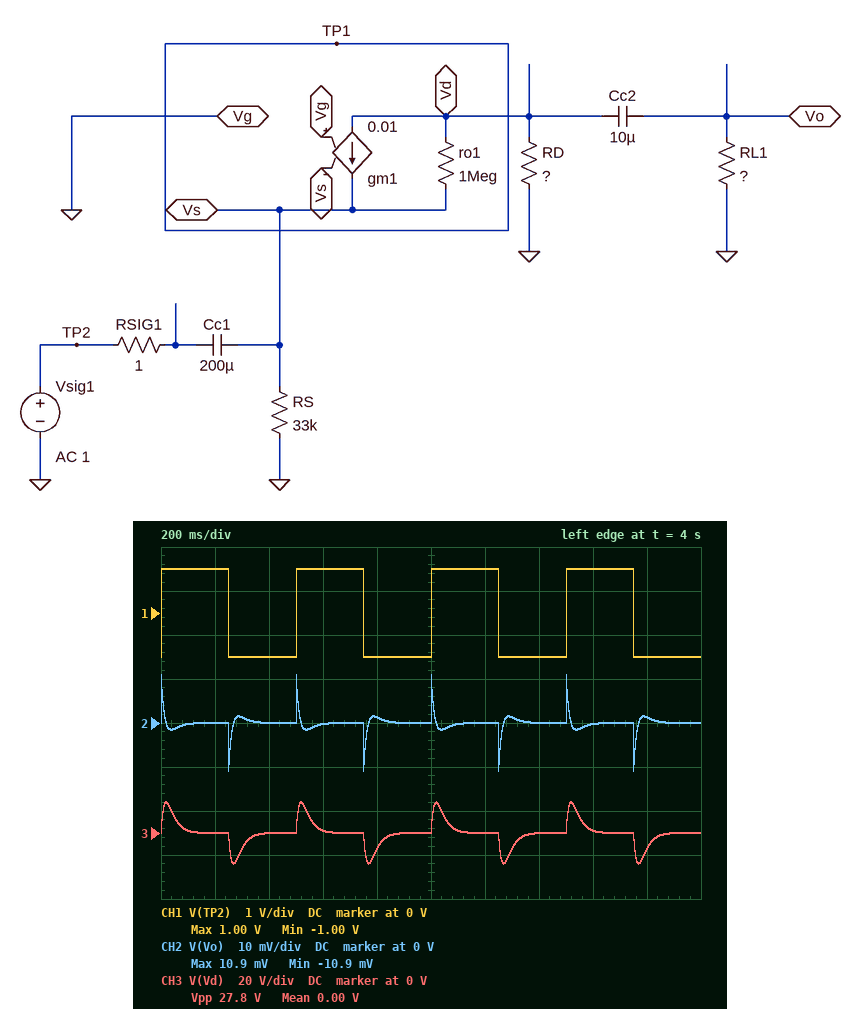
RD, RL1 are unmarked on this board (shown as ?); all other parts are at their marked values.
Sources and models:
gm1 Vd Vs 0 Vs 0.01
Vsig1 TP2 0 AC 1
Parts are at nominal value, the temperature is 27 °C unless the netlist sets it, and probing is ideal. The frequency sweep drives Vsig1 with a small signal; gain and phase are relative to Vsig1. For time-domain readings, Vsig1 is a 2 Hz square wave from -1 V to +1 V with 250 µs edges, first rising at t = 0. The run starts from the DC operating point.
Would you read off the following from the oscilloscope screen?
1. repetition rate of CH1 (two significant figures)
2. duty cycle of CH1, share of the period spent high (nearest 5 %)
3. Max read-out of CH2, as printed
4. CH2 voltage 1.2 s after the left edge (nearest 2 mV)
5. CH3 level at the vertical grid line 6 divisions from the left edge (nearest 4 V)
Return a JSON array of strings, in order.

["2.0 Hz", "50 %", "10.9 mV", "0 V", "0 V"]
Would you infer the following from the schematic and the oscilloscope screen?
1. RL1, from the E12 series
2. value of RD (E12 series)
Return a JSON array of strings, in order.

["0.56 Ω", "1.8 kΩ"]
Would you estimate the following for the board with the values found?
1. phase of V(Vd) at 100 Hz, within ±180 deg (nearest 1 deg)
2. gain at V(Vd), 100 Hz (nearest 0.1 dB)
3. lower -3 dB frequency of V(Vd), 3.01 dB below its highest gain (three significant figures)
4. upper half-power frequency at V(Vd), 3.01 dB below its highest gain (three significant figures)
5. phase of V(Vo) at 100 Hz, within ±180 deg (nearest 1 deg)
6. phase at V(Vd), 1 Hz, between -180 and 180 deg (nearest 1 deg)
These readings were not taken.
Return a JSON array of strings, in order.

["-80 deg", "3.9 dB", "3.46 Hz", "20.2 Hz", "10 deg", "76 deg"]
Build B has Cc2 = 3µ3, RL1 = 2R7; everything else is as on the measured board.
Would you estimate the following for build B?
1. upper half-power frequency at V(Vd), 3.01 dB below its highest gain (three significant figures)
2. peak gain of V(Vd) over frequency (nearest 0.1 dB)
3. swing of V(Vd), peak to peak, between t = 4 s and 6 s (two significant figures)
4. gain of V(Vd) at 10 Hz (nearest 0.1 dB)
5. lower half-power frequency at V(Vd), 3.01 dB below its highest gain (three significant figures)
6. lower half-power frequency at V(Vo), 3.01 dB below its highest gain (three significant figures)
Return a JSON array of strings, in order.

["40.0 Hz", "22.8 dB", "43 V", "22.3 dB", "5.29 Hz", "28.9 Hz"]
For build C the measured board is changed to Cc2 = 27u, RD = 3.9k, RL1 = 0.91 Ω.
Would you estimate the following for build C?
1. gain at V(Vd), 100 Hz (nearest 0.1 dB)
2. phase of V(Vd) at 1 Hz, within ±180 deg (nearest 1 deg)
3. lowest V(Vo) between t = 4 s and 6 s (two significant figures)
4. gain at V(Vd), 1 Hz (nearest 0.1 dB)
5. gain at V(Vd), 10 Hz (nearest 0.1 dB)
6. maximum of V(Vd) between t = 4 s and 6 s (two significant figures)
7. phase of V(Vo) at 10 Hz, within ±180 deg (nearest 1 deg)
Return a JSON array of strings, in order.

["-4.7 dB", "49 deg", "-18 mV", "12.1 dB", "13.1 dB", "8.9 V", "47 deg"]
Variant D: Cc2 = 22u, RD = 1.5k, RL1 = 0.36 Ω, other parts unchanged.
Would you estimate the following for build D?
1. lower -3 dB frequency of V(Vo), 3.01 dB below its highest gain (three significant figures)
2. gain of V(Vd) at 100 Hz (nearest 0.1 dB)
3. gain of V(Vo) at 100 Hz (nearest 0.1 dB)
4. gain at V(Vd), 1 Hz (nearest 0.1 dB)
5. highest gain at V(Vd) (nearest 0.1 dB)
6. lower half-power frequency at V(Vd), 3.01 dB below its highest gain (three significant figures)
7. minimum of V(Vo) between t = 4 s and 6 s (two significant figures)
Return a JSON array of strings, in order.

["10.0 Hz", "-2.9 dB", "-49.0 dB", "5.2 dB", "15.0 dB", "2.50 Hz", "-7.1 mV"]
